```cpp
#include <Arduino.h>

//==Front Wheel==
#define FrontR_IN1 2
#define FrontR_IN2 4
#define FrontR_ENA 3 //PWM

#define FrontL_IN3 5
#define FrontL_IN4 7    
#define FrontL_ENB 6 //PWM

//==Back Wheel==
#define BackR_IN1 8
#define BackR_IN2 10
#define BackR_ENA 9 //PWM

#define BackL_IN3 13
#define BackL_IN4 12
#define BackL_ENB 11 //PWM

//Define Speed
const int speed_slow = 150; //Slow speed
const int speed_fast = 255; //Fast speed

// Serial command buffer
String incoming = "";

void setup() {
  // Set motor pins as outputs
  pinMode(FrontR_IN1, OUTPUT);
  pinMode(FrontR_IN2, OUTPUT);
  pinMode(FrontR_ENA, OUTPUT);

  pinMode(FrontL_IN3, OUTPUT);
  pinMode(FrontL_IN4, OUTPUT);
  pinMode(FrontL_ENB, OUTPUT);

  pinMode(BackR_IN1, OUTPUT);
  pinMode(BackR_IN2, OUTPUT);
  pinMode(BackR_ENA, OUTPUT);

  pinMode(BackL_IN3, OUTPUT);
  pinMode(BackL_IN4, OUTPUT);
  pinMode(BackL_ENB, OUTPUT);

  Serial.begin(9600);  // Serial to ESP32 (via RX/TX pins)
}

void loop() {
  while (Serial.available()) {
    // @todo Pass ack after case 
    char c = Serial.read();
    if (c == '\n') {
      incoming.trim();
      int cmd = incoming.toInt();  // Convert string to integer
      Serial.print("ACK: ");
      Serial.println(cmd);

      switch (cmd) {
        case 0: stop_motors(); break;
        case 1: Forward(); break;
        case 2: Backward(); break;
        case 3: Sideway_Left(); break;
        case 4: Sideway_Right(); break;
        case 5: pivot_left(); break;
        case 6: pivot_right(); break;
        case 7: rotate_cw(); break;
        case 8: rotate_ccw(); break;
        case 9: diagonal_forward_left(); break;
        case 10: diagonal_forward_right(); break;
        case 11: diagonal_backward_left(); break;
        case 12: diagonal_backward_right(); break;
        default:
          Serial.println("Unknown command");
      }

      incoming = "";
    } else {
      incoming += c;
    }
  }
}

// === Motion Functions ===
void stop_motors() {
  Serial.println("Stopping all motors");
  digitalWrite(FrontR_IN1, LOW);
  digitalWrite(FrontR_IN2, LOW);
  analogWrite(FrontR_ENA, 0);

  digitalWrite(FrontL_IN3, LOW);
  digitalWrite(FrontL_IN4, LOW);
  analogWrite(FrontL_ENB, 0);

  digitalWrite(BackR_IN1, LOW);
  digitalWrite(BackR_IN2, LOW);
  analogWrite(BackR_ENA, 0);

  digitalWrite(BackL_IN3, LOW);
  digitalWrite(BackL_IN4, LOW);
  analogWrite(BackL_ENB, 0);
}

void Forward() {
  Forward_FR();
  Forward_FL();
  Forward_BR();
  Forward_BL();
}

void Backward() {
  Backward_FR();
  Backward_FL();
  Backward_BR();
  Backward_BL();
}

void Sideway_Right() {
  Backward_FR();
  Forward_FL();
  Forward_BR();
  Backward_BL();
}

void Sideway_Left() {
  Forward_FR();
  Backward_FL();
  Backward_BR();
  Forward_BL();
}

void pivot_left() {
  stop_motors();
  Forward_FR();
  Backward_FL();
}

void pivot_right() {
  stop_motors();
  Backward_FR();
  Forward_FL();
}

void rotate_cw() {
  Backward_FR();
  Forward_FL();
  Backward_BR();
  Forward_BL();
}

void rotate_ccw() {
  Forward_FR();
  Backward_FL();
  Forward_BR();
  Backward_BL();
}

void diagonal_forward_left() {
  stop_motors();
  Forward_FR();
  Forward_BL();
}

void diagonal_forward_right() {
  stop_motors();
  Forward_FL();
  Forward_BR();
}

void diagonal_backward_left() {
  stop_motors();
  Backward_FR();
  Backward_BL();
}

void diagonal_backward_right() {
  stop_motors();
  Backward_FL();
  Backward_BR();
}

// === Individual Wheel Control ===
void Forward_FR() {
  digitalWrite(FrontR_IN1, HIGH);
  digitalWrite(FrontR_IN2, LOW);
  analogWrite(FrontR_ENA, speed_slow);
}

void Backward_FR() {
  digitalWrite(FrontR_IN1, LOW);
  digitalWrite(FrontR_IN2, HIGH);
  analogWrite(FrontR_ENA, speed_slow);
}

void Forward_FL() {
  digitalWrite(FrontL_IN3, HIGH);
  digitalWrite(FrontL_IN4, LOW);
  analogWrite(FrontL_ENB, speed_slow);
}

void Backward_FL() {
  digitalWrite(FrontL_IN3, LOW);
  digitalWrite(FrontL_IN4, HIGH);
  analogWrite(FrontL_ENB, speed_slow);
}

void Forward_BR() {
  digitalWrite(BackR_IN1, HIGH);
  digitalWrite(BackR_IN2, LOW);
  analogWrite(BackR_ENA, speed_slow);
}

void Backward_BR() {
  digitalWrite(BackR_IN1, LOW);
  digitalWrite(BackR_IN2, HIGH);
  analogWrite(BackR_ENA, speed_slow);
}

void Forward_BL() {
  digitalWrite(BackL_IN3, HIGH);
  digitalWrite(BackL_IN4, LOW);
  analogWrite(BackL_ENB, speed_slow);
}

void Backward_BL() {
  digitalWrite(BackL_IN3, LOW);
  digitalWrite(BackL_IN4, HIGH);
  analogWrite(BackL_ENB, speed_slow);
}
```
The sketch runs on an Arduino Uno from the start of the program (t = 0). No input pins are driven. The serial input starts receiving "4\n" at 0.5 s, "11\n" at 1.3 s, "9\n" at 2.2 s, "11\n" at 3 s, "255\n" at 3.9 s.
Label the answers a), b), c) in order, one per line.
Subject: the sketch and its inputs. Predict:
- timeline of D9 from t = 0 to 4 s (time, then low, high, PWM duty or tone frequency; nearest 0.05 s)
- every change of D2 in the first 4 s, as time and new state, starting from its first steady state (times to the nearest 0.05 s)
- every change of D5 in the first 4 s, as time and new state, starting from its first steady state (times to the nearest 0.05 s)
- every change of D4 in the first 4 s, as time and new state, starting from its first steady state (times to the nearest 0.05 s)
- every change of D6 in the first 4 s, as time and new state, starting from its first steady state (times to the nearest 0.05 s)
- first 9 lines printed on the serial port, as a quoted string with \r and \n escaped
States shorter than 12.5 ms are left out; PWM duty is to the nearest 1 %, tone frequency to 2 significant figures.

a) 0 s low; 0.5 s PWM 59 %; 1.3 s low
b) 0 s low; 2.2 s high; 3 s low
c) 0 s low; 0.5 s high; 1.3 s low
d) 0 s low; 0.5 s high; 2.2 s low; 3 s high
e) 0 s low; 0.5 s PWM 59 %; 1.3 s low
f) "ACK: 4\r\nACK: 11\r\nStopping all motors\r\nACK: 9\r\nStopping all motors\r\nACK: 11\r\nStopping all motors\r\nACK: 255\r\nUnknown command\r\n"
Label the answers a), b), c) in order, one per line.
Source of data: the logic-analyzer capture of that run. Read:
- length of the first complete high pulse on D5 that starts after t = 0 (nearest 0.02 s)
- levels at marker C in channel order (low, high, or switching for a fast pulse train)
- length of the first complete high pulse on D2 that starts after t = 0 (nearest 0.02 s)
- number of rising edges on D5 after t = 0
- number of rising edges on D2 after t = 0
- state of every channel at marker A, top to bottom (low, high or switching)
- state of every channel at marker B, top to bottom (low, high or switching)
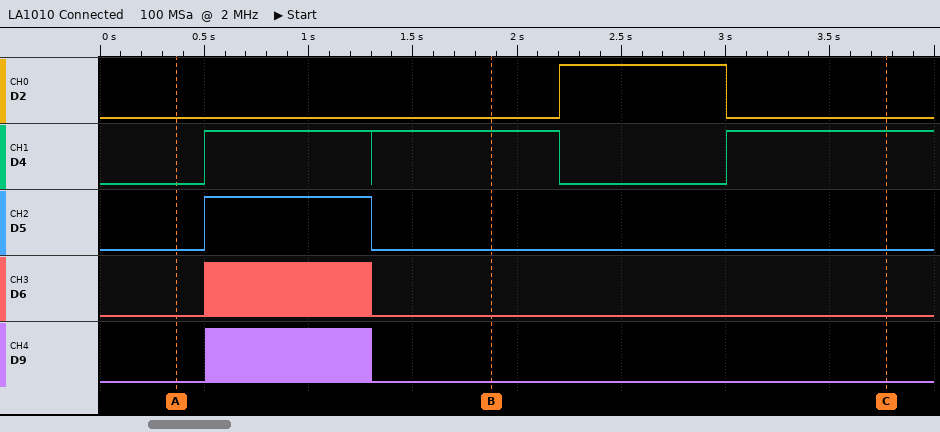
a) 0.80 s
b) D2 low, D4 high, D5 low, D6 low, D9 low
c) 0.80 s
d) 1
e) 1
f) D2 low, D4 low, D5 low, D6 low, D9 low
g) D2 low, D4 high, D5 low, D6 low, D9 low
